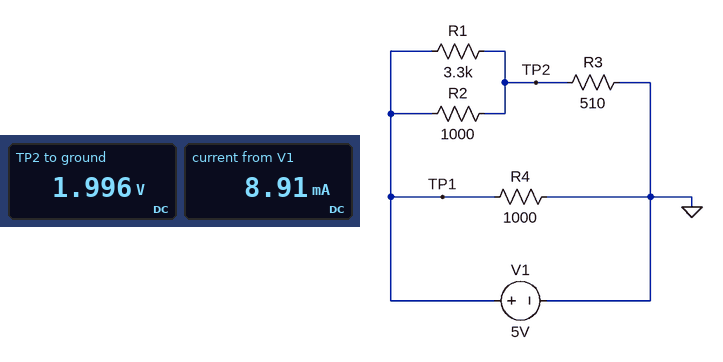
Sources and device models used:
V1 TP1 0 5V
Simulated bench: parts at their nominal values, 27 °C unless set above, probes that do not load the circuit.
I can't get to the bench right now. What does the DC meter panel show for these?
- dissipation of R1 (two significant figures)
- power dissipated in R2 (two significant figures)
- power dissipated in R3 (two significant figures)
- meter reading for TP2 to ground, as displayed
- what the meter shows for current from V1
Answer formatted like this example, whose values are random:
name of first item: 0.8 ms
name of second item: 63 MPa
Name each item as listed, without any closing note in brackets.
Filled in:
dissipation of R1: 2.7 mW
power dissipated in R2: 9.0 mW
power dissipated in R3: 7.8 mW
meter reading for TP2 to ground, as displayed: 1.996 V
what the meter shows for current from V1: 8.91 mA
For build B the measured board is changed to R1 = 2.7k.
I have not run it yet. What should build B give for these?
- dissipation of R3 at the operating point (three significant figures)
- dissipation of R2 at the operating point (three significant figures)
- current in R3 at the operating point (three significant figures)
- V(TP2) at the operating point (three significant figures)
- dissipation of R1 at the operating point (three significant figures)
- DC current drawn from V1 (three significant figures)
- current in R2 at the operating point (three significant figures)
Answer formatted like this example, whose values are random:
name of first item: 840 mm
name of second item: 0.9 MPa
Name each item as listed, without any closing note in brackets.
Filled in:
dissipation of R3 at the operating point: 8.30 mW
dissipation of R2 at the operating point: 8.66 mW
current in R3 at the operating point: 4.03 mA
V(TP2) at the operating point: 2.06 V
dissipation of R1 at the operating point: 3.21 mW
DC current drawn from V1: 9.03 mA
current in R2 at the operating point: 2.94 mA
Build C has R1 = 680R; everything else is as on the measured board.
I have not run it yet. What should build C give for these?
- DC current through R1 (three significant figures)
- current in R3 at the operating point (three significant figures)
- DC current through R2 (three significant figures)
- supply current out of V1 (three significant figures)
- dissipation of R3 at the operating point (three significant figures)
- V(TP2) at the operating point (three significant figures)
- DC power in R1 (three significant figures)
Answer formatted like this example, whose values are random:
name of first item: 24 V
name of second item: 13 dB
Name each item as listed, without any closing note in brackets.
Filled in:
DC current through R1: 3.25 mA
current in R3 at the operating point: 5.47 mA
DC current through R2: 2.21 mA
supply current out of V1: 10.5 mA
dissipation of R3 at the operating point: 15.2 mW
V(TP2) at the operating point: 2.79 V
DC power in R1: 7.20 mW
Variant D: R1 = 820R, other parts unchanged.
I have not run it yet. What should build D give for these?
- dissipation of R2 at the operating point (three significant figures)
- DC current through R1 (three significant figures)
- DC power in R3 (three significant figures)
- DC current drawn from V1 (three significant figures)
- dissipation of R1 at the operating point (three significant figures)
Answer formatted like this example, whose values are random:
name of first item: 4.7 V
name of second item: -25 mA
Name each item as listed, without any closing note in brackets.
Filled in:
dissipation of R2 at the operating point: 5.50 mW
DC current through R1: 2.86 mA
DC power in R3: 13.8 mW
DC current drawn from V1: 10.2 mA
dissipation of R1 at the operating point: 6.71 mW
